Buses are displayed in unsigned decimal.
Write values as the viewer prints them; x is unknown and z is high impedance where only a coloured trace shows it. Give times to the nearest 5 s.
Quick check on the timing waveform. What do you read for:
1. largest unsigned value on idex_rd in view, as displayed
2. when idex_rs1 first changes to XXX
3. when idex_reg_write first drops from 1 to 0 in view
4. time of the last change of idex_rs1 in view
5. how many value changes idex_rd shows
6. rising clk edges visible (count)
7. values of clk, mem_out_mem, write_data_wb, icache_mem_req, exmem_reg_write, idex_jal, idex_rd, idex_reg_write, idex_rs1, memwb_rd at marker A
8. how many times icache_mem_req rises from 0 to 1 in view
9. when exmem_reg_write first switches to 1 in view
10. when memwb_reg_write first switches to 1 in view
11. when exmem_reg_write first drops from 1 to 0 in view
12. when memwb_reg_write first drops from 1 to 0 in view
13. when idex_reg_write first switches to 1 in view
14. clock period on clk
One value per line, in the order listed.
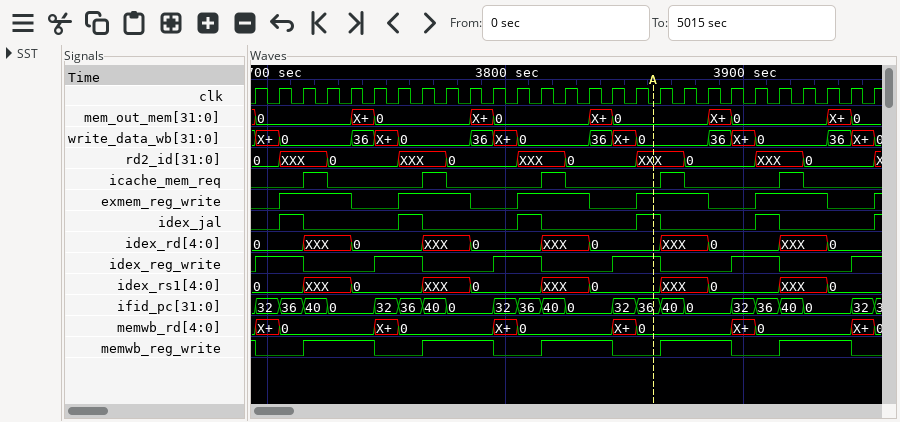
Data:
0
3715 s
3715 s
3935 s
10
27
clk=0, mem_out_mem=0, write_data_wb=0, icache_mem_req=0, exmem_reg_write=1, idex_jal=1, idex_rd=0, idex_reg_write=1, idex_rs1=0, memwb_rd=0
5
3705 s
3715 s
3735 s
3695 s
3695 s
10 s
